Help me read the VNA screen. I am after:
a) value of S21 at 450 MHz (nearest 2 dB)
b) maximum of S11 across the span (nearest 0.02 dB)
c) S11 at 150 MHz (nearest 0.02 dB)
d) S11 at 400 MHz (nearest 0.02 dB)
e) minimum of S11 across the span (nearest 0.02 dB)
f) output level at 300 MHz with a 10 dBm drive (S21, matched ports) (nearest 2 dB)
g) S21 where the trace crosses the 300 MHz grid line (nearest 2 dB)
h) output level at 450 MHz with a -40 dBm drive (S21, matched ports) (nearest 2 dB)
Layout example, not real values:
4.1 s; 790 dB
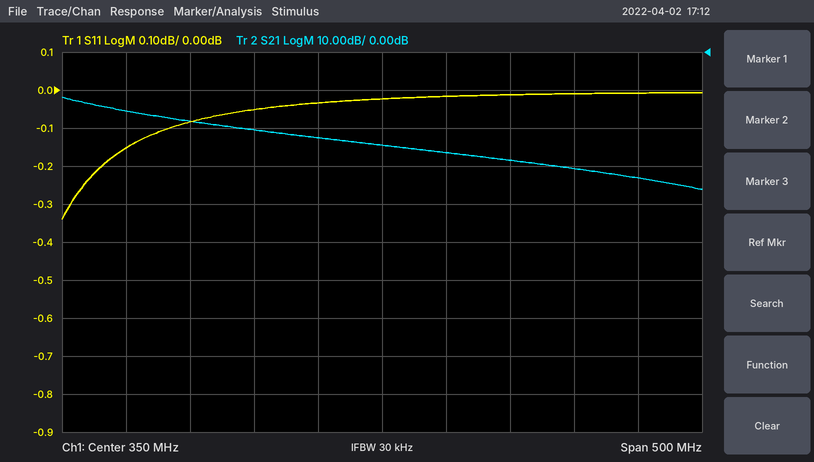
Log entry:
-28 dB; 0.00 dB; -0.16 dB; -0.02 dB; -0.34 dB; -12 dBm; -22 dB; -68 dBm
